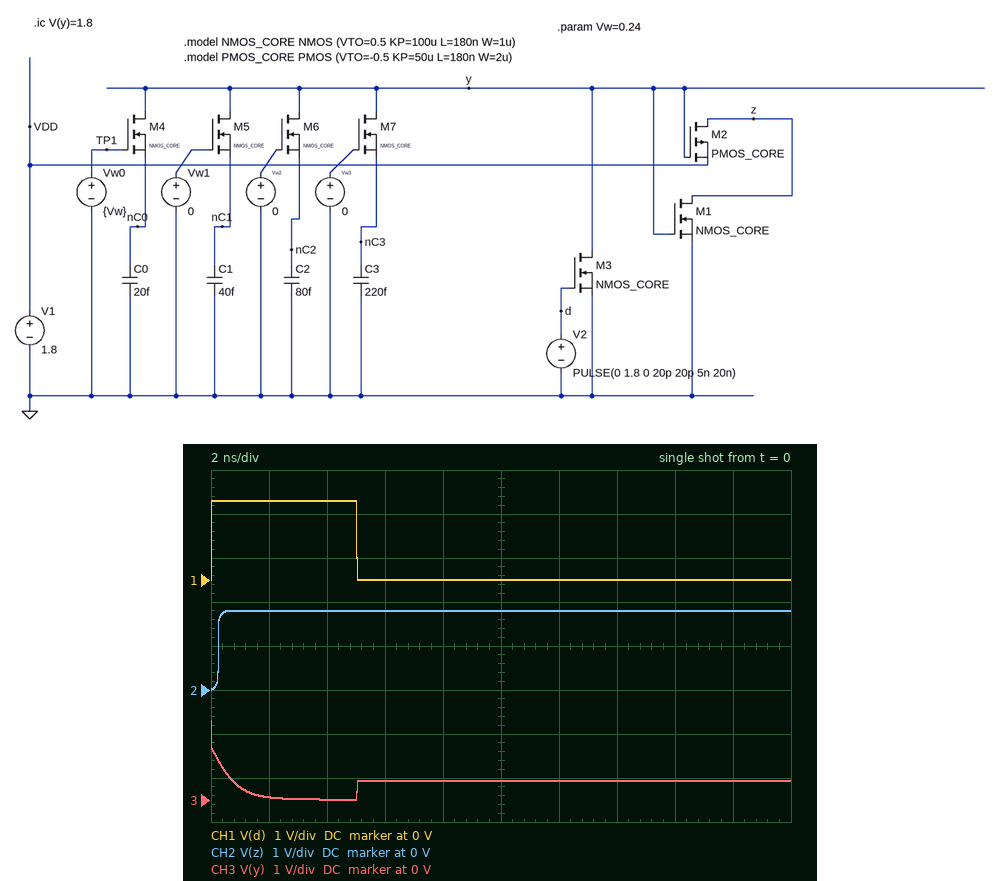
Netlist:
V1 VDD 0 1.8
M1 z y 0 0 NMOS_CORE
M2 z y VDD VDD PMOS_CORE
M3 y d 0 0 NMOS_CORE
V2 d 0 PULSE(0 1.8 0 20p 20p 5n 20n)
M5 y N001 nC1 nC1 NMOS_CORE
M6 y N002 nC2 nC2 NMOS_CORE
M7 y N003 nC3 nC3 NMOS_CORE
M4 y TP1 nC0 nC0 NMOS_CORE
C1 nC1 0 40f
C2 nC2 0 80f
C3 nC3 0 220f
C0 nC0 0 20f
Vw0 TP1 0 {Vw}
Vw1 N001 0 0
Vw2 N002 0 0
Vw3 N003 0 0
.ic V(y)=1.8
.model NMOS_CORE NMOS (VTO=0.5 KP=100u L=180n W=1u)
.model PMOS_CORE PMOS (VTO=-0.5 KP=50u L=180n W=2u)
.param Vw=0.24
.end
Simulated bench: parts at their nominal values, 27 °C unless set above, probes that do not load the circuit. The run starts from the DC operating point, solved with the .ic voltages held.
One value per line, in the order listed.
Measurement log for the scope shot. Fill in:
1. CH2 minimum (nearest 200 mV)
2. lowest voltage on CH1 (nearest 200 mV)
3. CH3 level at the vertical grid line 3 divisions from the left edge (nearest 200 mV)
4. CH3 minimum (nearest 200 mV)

0 V
0 V
400 mV
0 V
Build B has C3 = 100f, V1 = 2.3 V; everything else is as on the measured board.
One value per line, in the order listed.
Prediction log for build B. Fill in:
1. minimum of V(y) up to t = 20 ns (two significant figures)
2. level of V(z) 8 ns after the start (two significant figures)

3.0 mV
2.3 V
